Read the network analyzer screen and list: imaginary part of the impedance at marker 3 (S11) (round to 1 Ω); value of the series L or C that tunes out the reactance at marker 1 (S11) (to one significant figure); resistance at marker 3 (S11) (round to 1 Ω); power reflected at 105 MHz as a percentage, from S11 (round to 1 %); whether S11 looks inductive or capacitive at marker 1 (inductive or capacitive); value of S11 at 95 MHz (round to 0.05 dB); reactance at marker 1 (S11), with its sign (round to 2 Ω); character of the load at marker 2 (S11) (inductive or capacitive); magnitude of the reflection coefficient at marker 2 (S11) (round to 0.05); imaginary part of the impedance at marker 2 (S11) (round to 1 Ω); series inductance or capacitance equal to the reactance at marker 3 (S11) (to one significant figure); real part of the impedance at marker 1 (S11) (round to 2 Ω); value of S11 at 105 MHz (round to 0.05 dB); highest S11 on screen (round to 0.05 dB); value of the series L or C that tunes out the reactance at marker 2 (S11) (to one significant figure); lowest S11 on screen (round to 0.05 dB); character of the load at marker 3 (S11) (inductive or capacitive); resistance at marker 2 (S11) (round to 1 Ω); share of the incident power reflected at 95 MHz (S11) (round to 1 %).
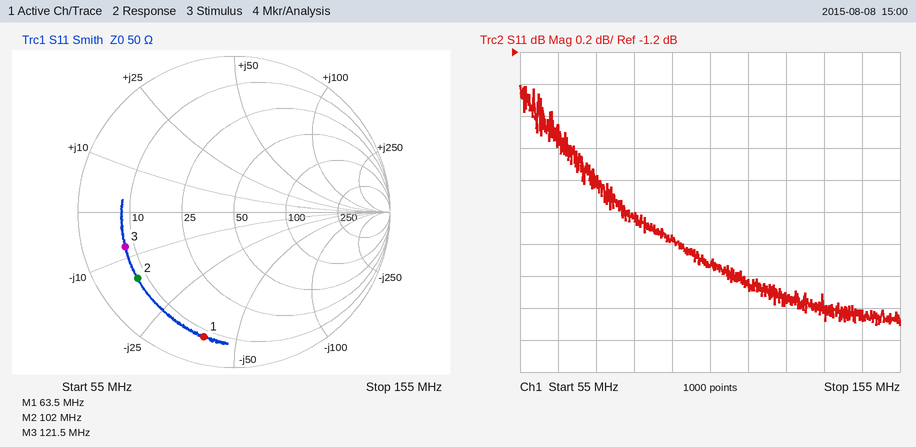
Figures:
-8 Ω
100 nH
8 Ω
56 %
capacitive
-2.35 dB
-38 Ω
capacitive
0.75
-15 Ω
200 pF
8 Ω
-2.55 dB
-1.40 dB
20 nH
-2.90 dB
capacitive
8 Ω
58 %
